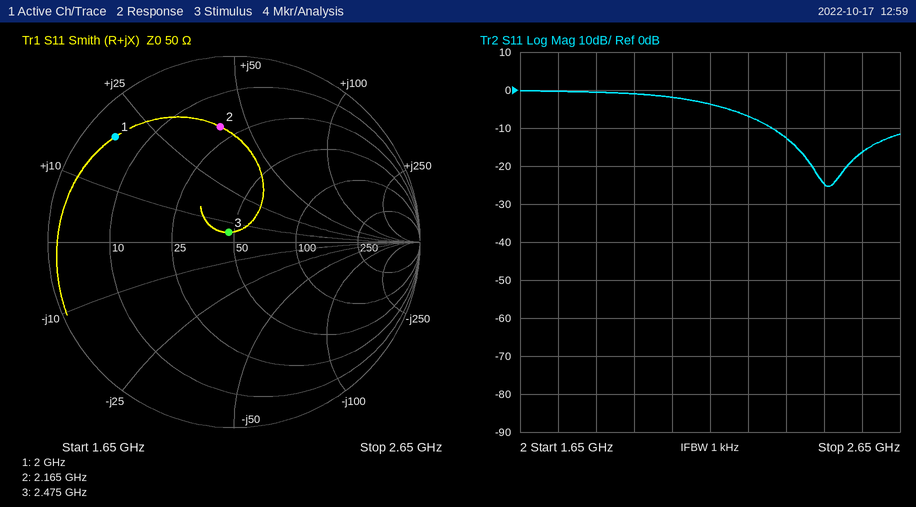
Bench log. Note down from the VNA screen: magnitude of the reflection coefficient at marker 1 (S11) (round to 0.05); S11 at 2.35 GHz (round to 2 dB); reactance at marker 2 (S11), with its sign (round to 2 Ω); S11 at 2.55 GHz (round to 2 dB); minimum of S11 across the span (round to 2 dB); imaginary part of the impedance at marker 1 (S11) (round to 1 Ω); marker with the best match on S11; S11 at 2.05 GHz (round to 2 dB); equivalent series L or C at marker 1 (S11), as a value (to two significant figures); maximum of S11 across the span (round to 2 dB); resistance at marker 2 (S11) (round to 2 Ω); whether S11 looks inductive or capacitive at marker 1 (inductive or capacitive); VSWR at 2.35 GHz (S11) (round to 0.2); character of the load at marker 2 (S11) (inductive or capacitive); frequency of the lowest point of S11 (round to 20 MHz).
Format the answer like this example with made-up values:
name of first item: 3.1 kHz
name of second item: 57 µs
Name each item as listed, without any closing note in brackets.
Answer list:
magnitude of the reflection coefficient at marker 1 (S11): 0.85
S11 at 2.35 GHz: -12 dB
reactance at marker 2 (S11), with its sign: +40 Ω
S11 at 2.55 GHz: -16 dB
minimum of S11 across the span: -26 dB
imaginary part of the impedance at marker 1 (S11): +19 Ω
marker with the best match on S11: marker 3
S11 at 2.05 GHz: -2 dB
equivalent series L or C at marker 1 (S11), as a value: 1.5 nH
maximum of S11 across the span: 0 dB
resistance at marker 2 (S11): 20 Ω
whether S11 looks inductive or capacitive at marker 1: inductive
VSWR at 2.35 GHz (S11): 1.6
character of the load at marker 2 (S11): inductive
frequency of the lowest point of S11: 2.46 GHz
